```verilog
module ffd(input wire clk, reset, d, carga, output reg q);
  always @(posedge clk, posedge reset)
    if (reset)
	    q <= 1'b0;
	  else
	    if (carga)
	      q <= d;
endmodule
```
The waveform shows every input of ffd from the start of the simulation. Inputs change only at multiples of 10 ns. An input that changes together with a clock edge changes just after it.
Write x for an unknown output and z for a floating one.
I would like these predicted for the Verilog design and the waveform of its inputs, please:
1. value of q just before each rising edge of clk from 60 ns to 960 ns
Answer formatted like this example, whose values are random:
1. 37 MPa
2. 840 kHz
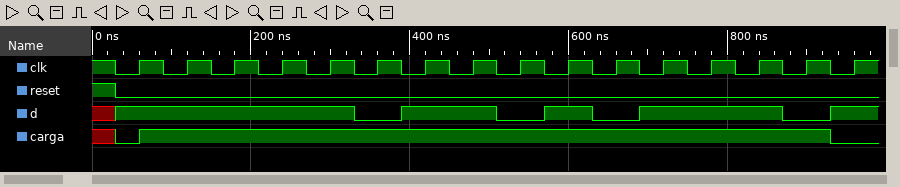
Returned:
1. 0 0 1 1 1 1 0 1 1 0 1 0 1 1 1 0
